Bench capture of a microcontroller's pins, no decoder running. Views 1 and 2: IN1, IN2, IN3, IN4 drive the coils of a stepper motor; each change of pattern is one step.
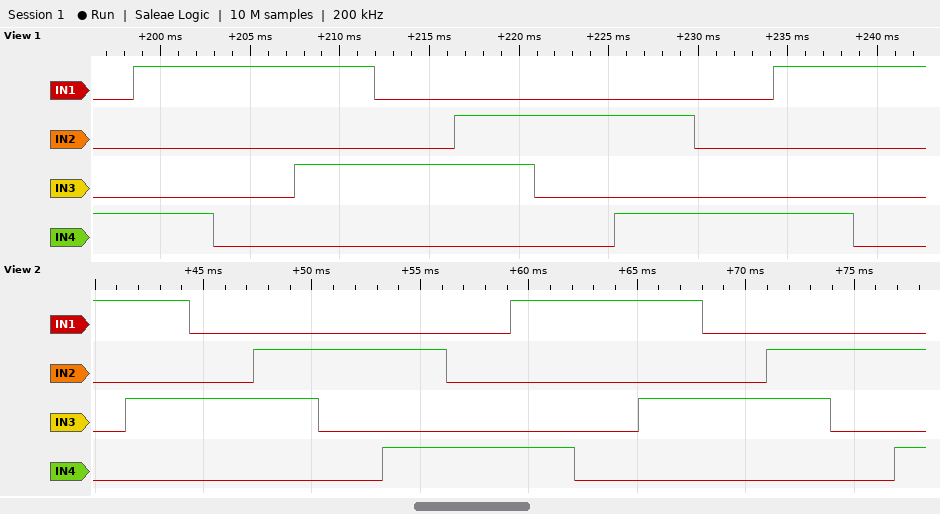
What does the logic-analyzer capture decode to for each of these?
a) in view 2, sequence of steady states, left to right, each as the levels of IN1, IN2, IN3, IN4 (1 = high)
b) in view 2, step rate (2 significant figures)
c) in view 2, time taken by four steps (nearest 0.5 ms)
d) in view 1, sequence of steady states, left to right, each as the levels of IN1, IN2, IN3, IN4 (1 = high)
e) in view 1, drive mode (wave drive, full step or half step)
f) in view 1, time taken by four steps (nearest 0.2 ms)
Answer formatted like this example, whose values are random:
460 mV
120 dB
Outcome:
1000 1010 0010 0110 0100 0101 0001 1001 1000 1010 0010 0110 0100 0101
340 steps/s
12.0 ms
0001 1001 1000 1010 0010 0110 0100 0101 0001 1001 1000
half step
18.0 ms
